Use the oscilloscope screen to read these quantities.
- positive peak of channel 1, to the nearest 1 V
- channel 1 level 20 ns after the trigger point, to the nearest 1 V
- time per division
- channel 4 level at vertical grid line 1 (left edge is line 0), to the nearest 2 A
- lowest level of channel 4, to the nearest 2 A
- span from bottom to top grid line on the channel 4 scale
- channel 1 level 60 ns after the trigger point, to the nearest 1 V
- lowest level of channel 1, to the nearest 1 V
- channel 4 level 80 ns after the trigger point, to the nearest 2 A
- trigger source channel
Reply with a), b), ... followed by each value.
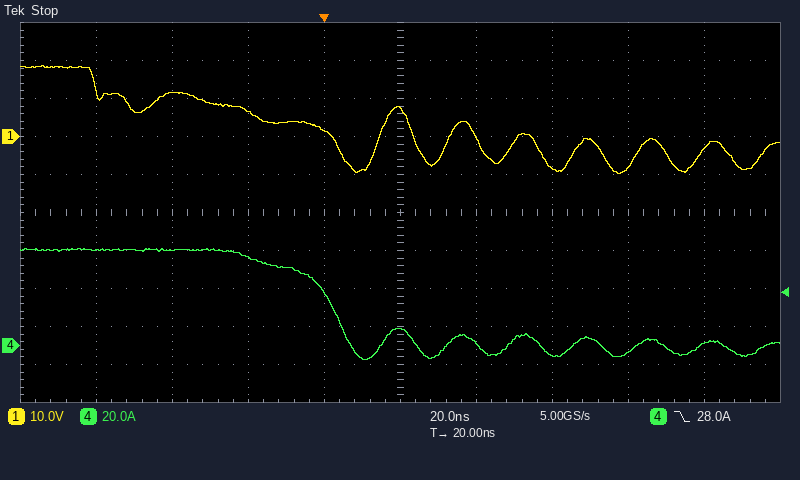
a) 19 V
b) 7 V
c) 20 ns
d) 50 A
e) -8 A
f) 200 A
g) -8 V
h) -10 V
i) -4 A
j) channel 4
